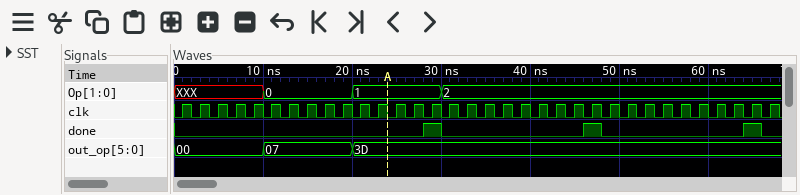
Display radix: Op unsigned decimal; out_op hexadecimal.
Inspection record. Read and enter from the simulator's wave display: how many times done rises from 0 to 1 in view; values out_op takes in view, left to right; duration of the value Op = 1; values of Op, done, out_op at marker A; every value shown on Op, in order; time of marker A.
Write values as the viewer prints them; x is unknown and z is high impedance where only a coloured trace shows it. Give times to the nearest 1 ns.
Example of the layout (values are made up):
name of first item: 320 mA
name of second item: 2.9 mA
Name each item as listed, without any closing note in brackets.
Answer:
how many times done rises from 0 to 1 in view: 3
values out_op takes in view, left to right: 00, 07, 3D
duration of the value Op = 1: 10 ns
values of Op, done, out_op at marker A: Op=1, done=0, out_op=3D
every value shown on Op, in order: XXX, 0, 1, 2
time of marker A: 24 ns
